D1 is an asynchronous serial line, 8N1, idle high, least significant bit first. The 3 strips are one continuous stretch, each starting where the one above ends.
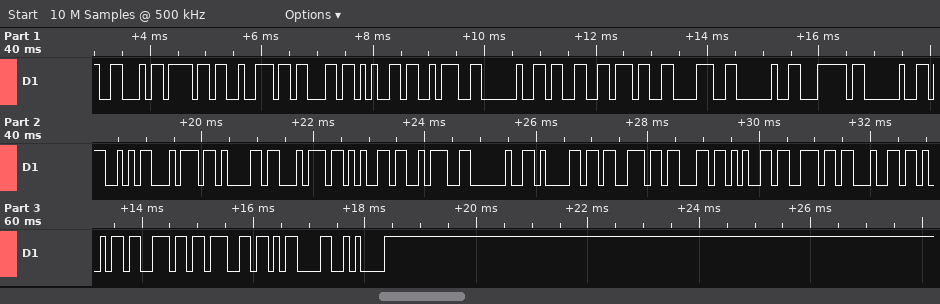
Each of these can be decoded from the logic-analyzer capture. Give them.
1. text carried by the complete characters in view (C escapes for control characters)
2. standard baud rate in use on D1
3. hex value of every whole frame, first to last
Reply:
"Force: 378 | State: ascending\r\n"
9600 baud
46 6F 72 63 65 3A 20 33 37 38 20 7C 20 53 74 61 74 65 3A 20 61 73 63 65 6E 64 69 6E 67 0D 0A
